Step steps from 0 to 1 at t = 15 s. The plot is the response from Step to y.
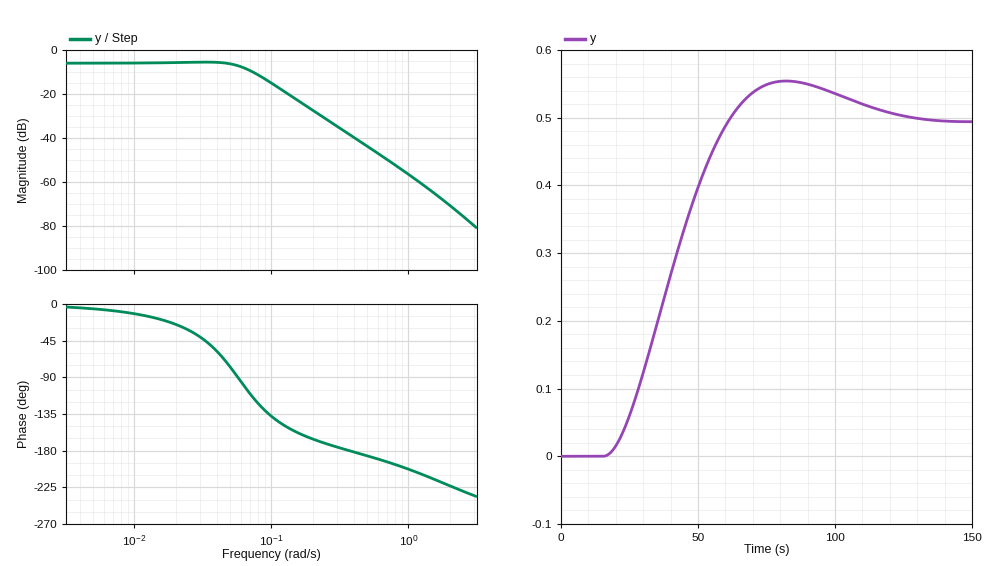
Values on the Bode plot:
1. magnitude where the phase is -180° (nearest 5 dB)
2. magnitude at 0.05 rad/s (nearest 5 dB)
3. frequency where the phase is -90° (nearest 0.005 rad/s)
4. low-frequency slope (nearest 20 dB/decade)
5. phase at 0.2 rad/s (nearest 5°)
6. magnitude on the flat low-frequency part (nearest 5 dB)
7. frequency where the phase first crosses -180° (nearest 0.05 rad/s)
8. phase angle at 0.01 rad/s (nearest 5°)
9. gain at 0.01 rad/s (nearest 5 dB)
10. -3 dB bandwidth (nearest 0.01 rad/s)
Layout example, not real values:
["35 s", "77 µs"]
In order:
["-40 dB", "-5 dB", "0.055 rad/s", "0 dB/decade", "-165°", "-5 dB", "0.35 rad/s", "-10°", "-5 dB", "0.07 rad/s"]
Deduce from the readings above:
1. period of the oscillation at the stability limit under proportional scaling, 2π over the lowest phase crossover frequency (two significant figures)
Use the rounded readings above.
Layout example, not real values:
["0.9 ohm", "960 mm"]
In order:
["18 s"]
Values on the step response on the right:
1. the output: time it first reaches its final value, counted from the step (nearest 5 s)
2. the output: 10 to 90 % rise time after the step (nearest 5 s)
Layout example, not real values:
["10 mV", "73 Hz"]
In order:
["45 s", "30 s"]
